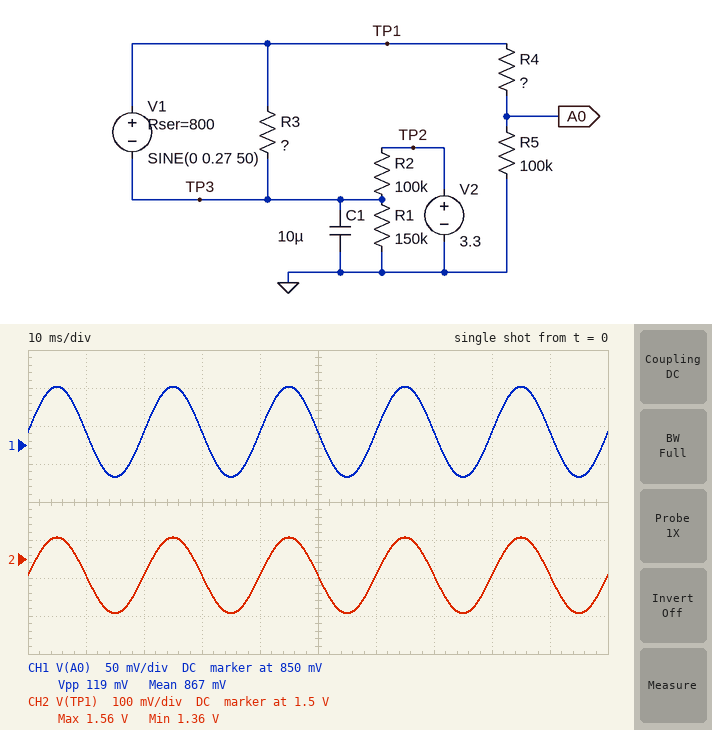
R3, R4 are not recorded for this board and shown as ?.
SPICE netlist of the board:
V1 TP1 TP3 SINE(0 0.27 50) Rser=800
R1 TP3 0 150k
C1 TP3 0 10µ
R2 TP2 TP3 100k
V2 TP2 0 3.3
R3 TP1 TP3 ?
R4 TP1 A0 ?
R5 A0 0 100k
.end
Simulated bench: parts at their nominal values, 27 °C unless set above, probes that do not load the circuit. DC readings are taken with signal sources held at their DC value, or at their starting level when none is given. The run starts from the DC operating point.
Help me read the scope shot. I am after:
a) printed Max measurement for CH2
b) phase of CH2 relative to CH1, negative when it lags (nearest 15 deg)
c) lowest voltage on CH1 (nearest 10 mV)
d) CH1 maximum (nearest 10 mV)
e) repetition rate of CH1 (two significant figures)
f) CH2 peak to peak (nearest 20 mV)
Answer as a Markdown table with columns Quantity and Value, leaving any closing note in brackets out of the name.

| Quantity | Value |
|---|---|
| printed Max measurement for CH2 | 1.56 V |
| phase of CH2 relative to CH1, negative when it lags | 0 deg |
| lowest voltage on CH1 | 810 mV |
| CH1 maximum | 930 mV |
| repetition rate of CH1 | 50 Hz |
| CH2 peak to peak | 200 mV |
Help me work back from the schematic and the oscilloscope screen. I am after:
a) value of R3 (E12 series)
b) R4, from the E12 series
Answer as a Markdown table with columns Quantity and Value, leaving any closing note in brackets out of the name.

| Quantity | Value |
|---|---|
| value of R3 | 470 Ω |
| R4, from the E12 series | 68 kΩ |
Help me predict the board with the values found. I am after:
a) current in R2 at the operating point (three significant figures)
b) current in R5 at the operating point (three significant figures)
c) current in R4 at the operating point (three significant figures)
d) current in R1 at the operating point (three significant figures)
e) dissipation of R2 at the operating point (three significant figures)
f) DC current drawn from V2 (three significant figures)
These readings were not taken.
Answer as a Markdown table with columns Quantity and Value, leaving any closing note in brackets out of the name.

| Quantity | Value |
|---|---|
| current in R2 at the operating point | 18.4 µA |
| current in R5 at the operating point | 8.67 µA |
| current in R4 at the operating point | 8.67 µA |
| current in R1 at the operating point | 9.73 µA |
| dissipation of R2 at the operating point | 33.9 µW |
| DC current drawn from V2 | 18.4 µA |
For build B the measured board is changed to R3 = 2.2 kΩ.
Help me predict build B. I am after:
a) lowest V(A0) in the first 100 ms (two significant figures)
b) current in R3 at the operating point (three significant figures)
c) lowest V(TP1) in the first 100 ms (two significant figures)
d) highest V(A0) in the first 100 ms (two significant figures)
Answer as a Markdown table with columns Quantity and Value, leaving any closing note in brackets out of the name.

| Quantity | Value |
|---|---|
| lowest V(A0) in the first 100 ms | 750 mV |
| current in R3 at the operating point | 2.31 µA |
| lowest V(TP1) in the first 100 ms | 1.3 V |
| highest V(A0) in the first 100 ms | 980 mV |
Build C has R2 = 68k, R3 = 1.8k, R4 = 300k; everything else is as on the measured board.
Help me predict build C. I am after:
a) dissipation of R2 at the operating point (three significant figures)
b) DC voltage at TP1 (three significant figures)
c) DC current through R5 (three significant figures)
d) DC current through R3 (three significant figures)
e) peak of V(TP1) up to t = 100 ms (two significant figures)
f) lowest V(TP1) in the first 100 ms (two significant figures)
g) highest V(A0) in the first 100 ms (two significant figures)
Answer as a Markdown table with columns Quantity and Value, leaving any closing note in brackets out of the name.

| Quantity | Value |
|---|---|
| dissipation of R2 at the operating point | 23.6 µW |
| DC voltage at TP1 | 2.03 V |
| DC current through R5 | 5.08 µA |
| DC current through R3 | 1.56 µA |
| peak of V(TP1) up to t = 100 ms | 2.2 V |
| lowest V(TP1) in the first 100 ms | 1.8 V |
| highest V(A0) in the first 100 ms | 550 mV |
